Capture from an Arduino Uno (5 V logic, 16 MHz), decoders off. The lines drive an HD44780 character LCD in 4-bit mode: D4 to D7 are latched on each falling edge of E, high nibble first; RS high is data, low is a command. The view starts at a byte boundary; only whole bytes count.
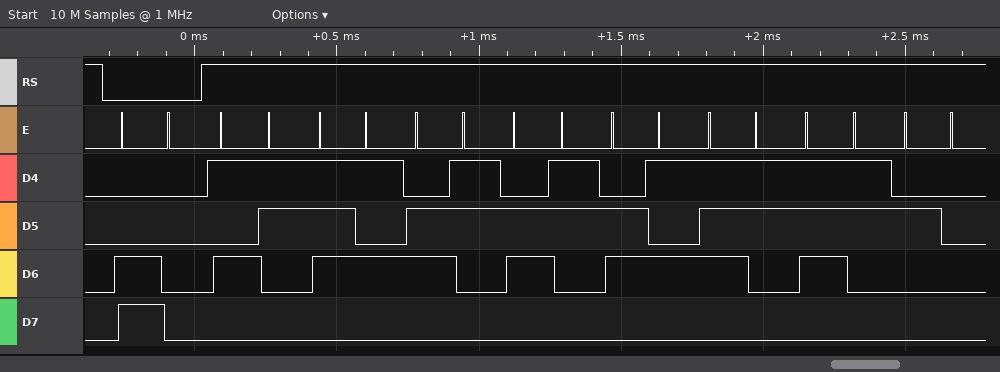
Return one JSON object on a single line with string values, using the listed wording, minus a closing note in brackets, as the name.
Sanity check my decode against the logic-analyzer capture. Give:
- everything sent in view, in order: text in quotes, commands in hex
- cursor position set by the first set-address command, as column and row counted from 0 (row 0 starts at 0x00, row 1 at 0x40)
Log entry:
{"everything sent in view, in order: text in quotes, commands in hex": "0xC0 \"Success \"", "cursor position set by the first set-address command, as column and row counted from 0": "column 0, row 1"}
